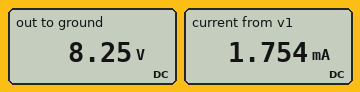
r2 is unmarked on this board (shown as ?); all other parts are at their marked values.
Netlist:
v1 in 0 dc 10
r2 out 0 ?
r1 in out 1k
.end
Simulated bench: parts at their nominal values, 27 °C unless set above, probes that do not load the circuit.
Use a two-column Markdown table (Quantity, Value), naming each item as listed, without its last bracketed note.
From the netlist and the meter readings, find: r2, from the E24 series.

| Quantity | Value |
|---|---|
| r2, from the E24 series | 4.7 kΩ |
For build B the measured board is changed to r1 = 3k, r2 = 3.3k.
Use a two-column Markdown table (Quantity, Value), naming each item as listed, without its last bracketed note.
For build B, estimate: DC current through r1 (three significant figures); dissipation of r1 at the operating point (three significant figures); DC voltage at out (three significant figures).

| Quantity | Value |
|---|---|
| DC current through r1 | 1.59 mA |
| dissipation of r1 at the operating point | 7.56 mW |
| DC voltage at out | 5.24 V |
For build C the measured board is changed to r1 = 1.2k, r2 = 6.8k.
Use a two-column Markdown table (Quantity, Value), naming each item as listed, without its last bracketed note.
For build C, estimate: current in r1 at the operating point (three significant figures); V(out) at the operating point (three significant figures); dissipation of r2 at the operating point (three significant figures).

| Quantity | Value |
|---|---|
| current in r1 at the operating point | 1.25 mA |
| V(out) at the operating point | 8.50 V |
| dissipation of r2 at the operating point | 10.6 mW |
